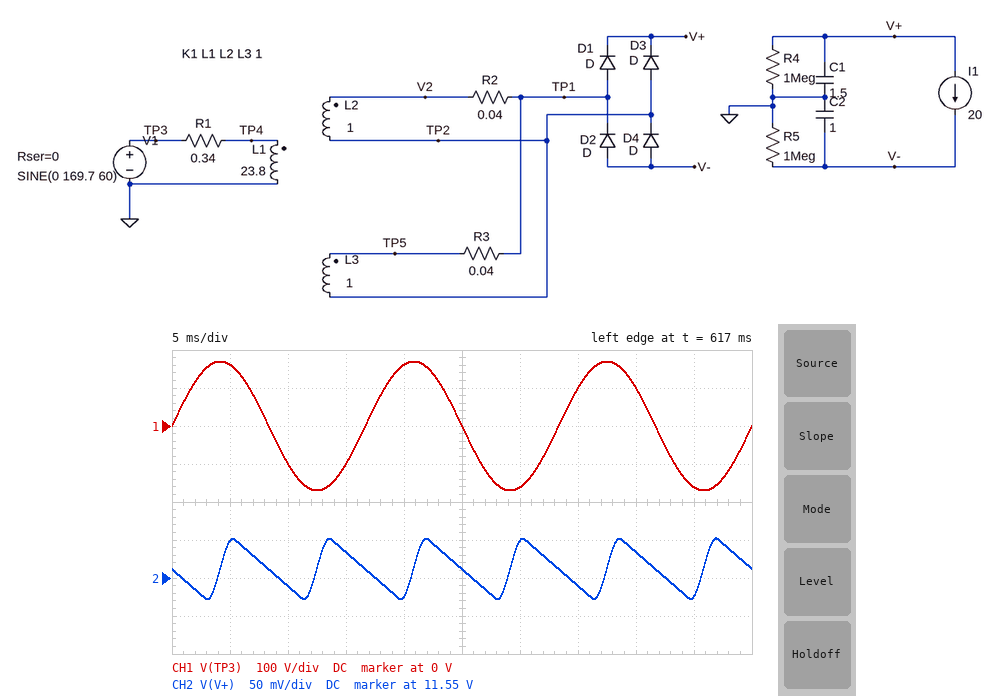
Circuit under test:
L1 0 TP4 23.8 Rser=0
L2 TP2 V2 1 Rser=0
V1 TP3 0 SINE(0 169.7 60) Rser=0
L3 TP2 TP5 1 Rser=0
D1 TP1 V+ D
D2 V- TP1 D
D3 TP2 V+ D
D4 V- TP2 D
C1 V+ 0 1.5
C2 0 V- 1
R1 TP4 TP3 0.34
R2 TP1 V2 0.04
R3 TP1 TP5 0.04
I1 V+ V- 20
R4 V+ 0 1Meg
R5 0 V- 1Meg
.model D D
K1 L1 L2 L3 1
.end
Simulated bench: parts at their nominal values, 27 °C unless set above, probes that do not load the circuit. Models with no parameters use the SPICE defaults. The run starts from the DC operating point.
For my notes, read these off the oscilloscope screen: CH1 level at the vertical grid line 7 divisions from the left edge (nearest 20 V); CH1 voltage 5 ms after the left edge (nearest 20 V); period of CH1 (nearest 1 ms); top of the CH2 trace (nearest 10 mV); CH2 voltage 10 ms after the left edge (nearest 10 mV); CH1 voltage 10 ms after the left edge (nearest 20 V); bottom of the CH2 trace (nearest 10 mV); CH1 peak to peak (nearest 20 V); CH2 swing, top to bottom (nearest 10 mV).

100 V
160 V
17 ms
11.60 V
11.54 V
-100 V
11.52 V
340 V
80 mV
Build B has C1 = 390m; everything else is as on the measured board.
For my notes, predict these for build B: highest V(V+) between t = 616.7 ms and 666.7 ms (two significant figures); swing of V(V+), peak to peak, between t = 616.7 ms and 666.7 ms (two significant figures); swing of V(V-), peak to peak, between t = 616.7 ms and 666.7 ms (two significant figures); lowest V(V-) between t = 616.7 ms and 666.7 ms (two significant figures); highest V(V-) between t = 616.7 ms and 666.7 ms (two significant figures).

22 V
310 mV
120 mV
-7.9 V
-7.8 V
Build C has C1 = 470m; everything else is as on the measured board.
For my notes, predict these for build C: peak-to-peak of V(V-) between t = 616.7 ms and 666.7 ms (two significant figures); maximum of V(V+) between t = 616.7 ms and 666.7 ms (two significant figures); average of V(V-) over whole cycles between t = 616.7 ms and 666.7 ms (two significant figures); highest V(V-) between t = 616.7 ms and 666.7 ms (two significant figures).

120 mV
20 V
-9.1 V
-9.0 V
